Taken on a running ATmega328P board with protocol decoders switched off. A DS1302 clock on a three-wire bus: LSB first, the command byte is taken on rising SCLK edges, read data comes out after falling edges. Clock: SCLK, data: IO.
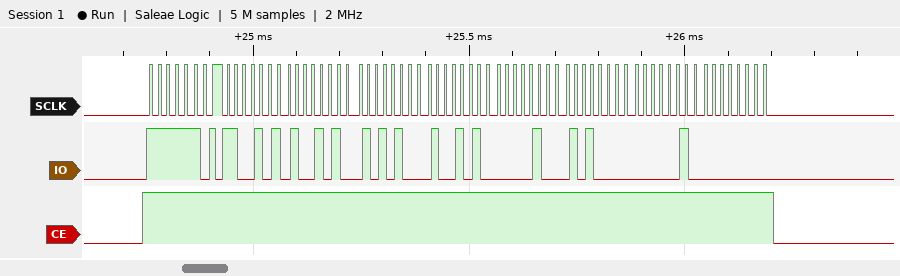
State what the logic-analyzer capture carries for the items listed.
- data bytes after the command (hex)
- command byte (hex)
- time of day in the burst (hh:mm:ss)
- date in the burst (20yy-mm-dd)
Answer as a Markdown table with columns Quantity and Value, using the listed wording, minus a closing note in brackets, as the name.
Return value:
| Quantity | Value |
|---|---|
| data bytes after the command | 53 29 15 29 10 05 20 00 |
| command byte | 0xBF |
| time of day in the burst | 15:29:53 |
| date in the burst | 2020-10-29 |
